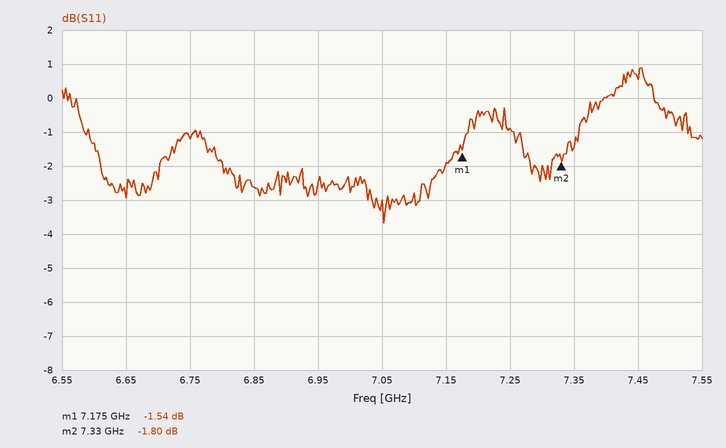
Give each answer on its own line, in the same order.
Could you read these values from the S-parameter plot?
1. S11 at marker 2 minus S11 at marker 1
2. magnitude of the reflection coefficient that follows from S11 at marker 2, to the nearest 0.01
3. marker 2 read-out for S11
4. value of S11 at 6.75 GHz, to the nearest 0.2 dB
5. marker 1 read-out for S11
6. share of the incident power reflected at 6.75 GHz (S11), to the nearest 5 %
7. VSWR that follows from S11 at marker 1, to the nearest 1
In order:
-0.26 dB
0.81
-1.80 dB
-1.2 dB
-1.54 dB
75 %
11
